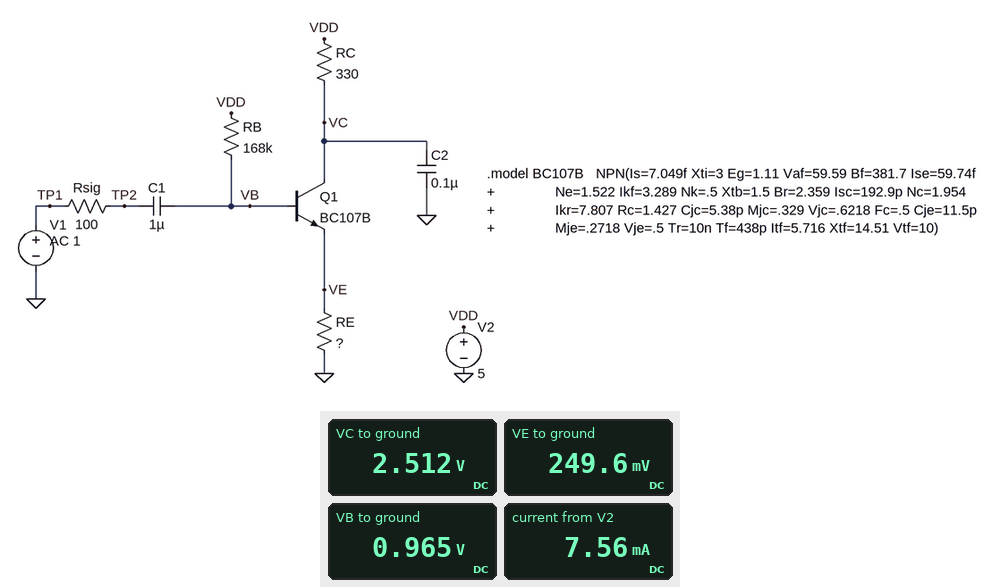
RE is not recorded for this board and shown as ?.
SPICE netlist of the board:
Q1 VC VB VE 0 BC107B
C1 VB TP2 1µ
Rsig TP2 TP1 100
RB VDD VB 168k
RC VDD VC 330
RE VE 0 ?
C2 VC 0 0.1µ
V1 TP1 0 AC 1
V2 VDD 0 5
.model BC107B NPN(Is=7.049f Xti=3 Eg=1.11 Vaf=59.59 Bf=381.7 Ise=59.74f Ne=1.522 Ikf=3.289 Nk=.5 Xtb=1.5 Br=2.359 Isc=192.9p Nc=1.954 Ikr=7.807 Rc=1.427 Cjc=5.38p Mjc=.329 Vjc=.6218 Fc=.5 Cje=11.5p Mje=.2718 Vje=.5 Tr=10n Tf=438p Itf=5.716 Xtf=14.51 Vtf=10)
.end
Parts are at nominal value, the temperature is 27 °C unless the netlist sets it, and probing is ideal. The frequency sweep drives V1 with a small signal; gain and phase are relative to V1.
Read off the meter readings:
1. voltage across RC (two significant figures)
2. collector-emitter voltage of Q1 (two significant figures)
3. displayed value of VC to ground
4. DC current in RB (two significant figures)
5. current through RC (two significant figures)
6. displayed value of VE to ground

2.5 V
2.3 V
2.512 V
24 µA
7.5 mA
249.6 mV
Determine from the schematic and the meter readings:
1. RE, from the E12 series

33 Ω
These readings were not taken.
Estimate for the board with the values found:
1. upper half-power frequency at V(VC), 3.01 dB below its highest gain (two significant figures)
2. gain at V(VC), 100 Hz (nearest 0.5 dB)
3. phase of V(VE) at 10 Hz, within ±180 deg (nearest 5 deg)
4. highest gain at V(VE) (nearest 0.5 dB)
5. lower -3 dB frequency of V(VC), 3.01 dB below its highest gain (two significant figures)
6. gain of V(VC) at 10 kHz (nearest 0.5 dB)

4.9 kHz
19.0 dB
55 deg
-1.0 dB
14 Hz
12.0 dB
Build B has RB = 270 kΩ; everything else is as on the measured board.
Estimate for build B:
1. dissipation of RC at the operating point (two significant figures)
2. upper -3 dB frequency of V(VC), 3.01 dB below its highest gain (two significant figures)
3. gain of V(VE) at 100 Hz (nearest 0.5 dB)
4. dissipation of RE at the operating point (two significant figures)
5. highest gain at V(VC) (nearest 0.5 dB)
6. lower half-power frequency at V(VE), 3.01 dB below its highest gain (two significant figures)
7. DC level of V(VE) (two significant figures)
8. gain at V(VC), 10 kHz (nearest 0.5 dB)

7.4 mW
4.9 kHz
-1.5 dB
740 µW
18.5 dB
13 Hz
160 mV
11.5 dB
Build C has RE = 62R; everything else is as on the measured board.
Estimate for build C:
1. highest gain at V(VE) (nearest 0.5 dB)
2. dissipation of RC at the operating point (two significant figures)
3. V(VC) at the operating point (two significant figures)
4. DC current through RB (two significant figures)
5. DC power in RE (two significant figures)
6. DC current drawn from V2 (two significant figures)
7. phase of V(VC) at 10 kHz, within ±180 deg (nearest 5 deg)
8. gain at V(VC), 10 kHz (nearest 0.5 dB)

-0.5 dB
17 mW
2.6 V
23 µA
3.2 mW
7.2 mA
115 deg
6.5 dB
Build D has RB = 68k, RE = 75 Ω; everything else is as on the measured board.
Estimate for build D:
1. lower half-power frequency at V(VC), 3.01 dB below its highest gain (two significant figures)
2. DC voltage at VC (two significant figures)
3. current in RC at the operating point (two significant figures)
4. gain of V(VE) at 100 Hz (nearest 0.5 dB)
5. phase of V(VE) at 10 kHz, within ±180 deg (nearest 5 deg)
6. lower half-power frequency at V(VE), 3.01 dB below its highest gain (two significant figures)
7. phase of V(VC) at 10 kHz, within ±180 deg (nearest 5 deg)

200 Hz
1.1 V
12 mA
-8.5 dB
5 deg
250 Hz
120 deg
